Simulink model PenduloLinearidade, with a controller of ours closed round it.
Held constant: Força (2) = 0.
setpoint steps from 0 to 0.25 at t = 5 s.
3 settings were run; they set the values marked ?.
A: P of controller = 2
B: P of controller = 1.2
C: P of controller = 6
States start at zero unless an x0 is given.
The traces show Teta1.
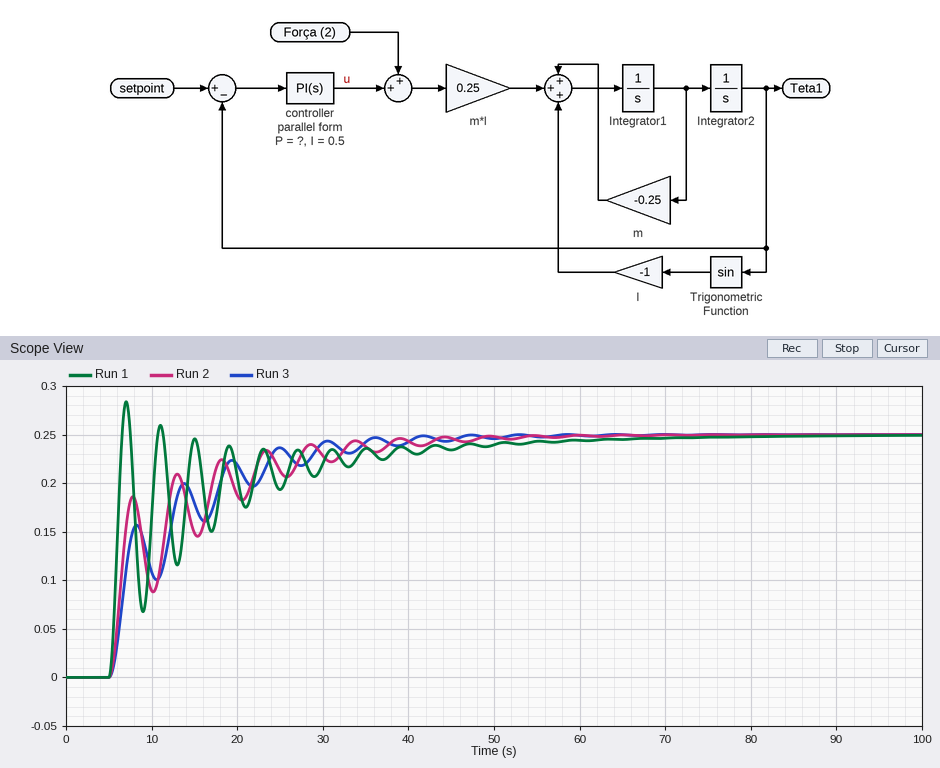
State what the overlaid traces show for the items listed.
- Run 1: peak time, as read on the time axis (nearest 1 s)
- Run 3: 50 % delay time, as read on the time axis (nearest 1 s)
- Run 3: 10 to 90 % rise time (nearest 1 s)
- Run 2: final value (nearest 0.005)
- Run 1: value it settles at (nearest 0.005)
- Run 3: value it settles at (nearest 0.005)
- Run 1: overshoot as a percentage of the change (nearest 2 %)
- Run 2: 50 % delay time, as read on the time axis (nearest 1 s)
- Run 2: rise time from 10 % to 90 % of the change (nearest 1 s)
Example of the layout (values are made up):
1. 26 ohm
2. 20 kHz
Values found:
1. 7 s
2. 7 s
3. 18 s
4. 0.250
5. 0.250
6. 0.250
7. 14 %
8. 7 s
9. 17 s
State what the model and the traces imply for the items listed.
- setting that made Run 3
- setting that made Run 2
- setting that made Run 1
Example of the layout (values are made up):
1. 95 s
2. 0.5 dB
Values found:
1. B
2. A
3. C
